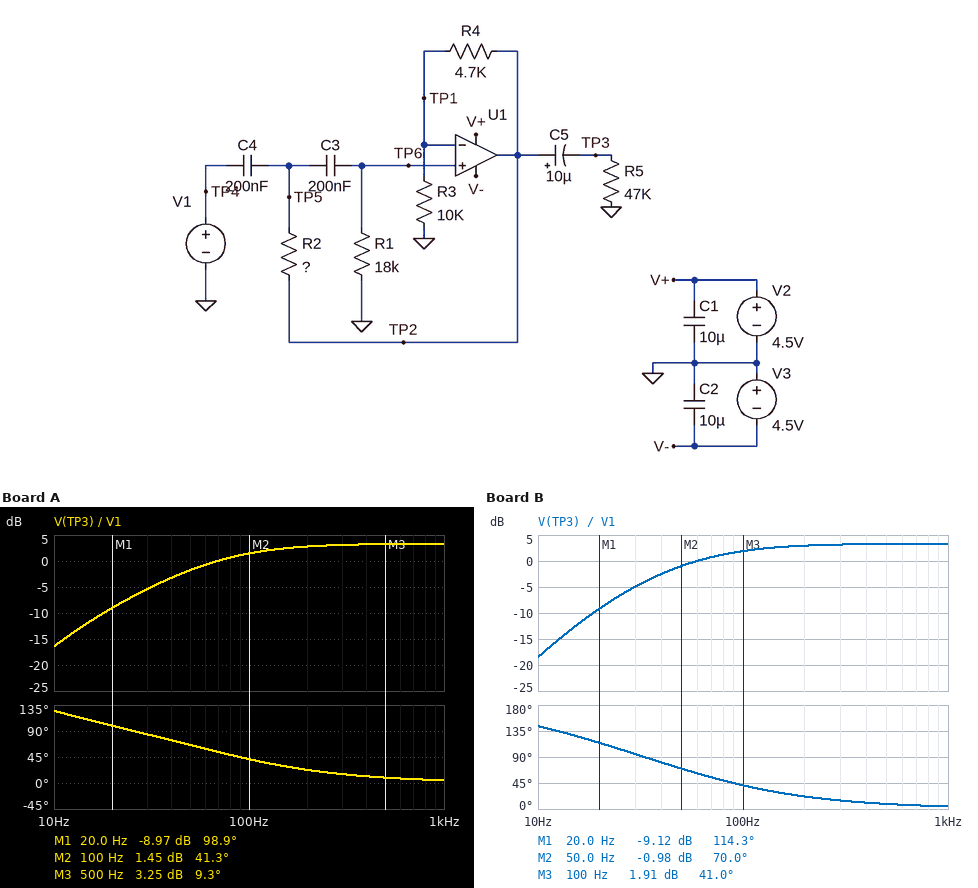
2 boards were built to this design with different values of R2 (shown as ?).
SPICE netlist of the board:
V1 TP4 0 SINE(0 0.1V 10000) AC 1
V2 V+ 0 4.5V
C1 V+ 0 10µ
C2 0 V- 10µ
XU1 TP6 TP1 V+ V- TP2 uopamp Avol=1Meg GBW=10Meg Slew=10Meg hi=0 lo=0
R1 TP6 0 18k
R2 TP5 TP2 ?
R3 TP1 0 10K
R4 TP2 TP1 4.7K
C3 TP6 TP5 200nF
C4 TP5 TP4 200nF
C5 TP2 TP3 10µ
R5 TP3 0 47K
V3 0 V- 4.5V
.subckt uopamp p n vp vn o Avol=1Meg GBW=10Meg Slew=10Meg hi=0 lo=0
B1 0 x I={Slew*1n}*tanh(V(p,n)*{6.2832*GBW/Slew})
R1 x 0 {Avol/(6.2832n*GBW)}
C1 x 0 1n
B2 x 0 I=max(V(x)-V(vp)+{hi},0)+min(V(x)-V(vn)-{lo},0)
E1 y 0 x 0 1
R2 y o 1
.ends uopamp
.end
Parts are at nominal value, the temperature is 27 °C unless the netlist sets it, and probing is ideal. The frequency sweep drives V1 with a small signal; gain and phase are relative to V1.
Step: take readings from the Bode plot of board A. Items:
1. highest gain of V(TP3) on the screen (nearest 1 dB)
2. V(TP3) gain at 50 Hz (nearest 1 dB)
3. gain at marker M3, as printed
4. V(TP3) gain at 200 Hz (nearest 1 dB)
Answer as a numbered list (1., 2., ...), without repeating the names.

1. 3 dB
2. -2 dB
3. 3.25 dB
4. 3 dB
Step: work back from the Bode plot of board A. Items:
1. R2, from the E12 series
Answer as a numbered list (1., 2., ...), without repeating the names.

1. 56 kΩ
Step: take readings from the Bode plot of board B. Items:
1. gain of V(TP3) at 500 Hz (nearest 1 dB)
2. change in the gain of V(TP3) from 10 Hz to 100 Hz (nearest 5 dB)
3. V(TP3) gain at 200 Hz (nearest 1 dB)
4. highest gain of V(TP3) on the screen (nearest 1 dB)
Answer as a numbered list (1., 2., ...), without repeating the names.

1. 3 dB
2. 20 dB
3. 3 dB
4. 3 dB
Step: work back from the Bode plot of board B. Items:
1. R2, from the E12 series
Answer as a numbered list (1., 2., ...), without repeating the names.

1. 33 kΩ
